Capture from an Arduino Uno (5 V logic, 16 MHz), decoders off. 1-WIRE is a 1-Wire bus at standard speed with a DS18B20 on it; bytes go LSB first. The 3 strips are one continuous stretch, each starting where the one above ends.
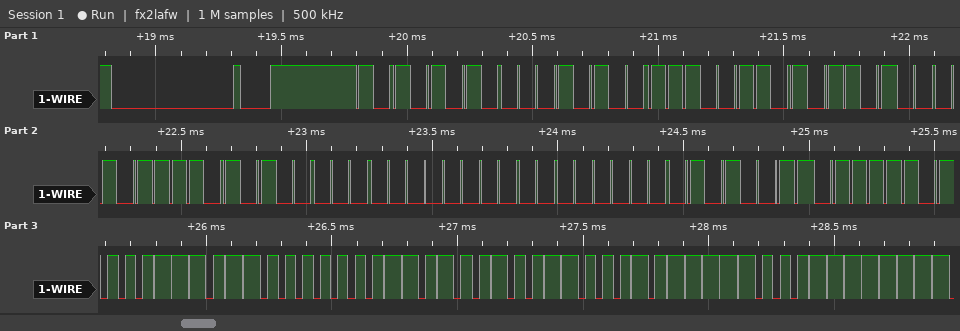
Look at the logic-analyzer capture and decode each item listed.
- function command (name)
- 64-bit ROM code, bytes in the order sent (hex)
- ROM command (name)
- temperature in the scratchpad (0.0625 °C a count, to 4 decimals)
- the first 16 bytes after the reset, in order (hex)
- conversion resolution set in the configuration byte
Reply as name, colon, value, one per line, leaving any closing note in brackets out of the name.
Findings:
function command: Read Scratchpad
64-bit ROM code, bytes in the order sent: 28 67 2D 7A 05 00 00 CA
ROM command: Match ROM
temperature in the scratchpad: 27.5000 °C
the first 16 bytes after the reset, in order: 55 28 67 2D 7A 05 00 00 CA BE B8 01 4B 46 1F FF
conversion resolution set in the configuration byte: 9 bits
